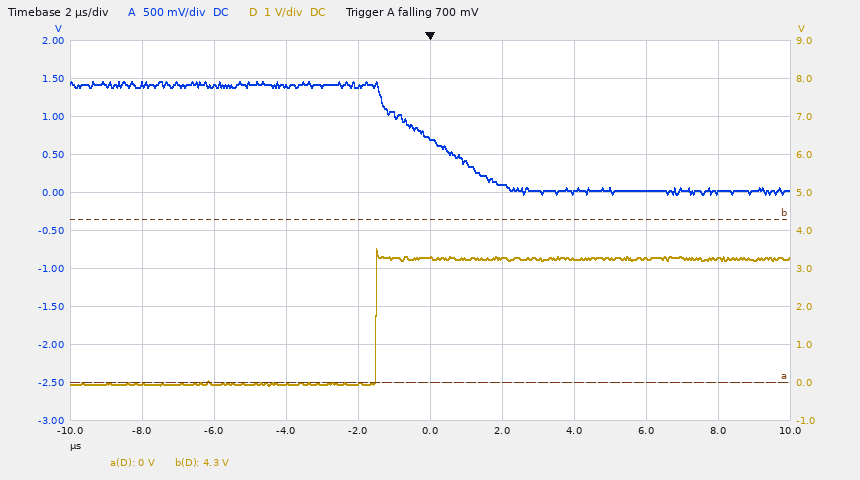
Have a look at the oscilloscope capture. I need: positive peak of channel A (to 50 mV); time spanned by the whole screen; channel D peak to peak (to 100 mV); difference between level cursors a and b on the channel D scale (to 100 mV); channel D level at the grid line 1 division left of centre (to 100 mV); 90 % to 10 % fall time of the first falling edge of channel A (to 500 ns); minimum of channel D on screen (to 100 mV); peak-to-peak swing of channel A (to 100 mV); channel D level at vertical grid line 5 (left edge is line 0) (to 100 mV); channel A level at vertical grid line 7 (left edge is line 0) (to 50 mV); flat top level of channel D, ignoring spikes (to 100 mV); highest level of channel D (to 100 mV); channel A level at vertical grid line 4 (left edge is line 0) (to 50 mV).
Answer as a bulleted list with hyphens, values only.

- 1.45 V
- 20 µs
- 3.6 V
- 4.3 V
- 0.0 V
- 3.0 µs
- -100 mV
- 1.50 V
- 3.3 V
- 0 mV
- 3.3 V
- 3.5 V
- 1.40 V
